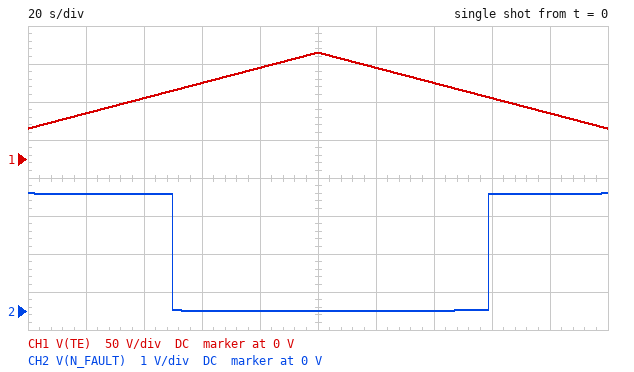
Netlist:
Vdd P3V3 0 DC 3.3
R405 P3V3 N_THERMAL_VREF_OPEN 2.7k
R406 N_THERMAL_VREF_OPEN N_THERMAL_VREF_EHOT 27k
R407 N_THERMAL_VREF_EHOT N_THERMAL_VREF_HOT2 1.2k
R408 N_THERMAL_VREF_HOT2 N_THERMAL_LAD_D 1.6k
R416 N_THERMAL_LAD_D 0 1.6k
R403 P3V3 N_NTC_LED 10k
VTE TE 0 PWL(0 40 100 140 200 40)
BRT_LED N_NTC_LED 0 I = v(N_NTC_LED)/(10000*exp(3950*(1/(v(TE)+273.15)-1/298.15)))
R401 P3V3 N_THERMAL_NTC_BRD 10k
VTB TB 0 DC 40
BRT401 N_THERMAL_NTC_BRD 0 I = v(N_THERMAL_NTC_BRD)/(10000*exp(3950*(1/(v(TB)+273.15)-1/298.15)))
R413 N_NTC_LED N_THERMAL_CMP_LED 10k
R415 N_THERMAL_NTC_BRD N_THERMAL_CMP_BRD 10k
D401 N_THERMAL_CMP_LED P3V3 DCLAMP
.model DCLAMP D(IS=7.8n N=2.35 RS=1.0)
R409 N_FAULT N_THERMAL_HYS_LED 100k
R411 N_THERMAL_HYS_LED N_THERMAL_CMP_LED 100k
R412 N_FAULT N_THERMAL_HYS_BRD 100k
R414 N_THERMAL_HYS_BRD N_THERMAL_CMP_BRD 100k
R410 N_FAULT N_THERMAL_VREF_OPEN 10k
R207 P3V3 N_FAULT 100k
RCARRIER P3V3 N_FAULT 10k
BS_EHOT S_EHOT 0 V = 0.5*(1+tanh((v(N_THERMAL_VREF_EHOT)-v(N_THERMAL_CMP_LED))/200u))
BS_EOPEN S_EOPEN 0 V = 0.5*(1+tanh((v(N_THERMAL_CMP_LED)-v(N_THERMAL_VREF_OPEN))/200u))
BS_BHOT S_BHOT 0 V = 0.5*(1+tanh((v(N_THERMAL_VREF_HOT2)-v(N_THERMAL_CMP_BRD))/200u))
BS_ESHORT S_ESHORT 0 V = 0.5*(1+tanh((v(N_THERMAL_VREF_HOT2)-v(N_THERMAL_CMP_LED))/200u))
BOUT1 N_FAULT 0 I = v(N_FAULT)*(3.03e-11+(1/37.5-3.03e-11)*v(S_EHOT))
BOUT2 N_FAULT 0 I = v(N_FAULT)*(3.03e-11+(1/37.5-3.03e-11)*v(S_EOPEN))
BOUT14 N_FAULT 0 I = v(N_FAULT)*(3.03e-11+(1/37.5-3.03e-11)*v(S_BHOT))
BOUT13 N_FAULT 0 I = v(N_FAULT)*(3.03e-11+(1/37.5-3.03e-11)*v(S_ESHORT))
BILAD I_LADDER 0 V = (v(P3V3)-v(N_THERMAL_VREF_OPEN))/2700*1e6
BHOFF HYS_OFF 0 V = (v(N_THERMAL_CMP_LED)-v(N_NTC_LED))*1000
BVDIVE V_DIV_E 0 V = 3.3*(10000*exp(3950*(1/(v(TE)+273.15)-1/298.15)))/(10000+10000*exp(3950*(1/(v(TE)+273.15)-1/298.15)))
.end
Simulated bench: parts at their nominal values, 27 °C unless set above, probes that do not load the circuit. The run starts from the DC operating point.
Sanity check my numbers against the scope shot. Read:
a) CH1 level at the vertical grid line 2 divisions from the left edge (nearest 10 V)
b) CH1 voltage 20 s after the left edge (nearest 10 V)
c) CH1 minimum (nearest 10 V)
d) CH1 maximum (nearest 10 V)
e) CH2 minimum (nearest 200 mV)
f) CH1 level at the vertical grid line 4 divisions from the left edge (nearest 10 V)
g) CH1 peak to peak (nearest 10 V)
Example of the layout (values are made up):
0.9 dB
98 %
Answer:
80 V
60 V
40 V
140 V
0 V
120 V
100 V
